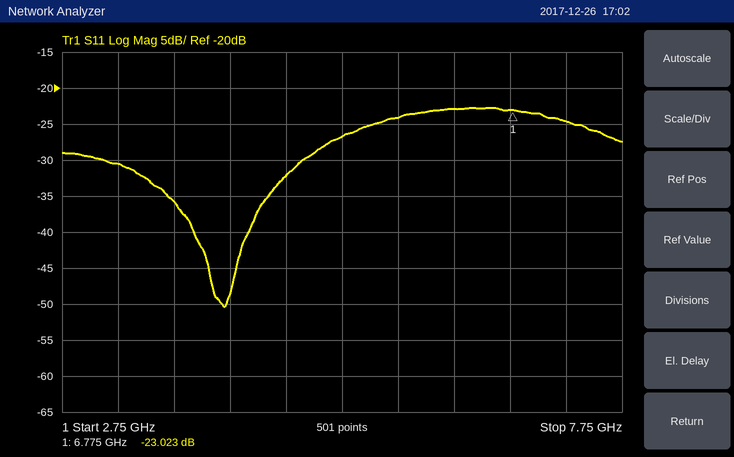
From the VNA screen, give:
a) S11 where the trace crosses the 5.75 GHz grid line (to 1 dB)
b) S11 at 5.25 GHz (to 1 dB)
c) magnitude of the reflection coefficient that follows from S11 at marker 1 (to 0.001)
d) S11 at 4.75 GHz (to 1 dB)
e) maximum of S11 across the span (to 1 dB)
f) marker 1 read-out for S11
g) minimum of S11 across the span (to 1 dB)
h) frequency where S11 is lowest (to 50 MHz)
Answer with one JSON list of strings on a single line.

["-24 dB", "-27 dB", "0.071", "-32 dB", "-23 dB", "-23.023 dB", "-50 dB", "4.20 GHz"]
